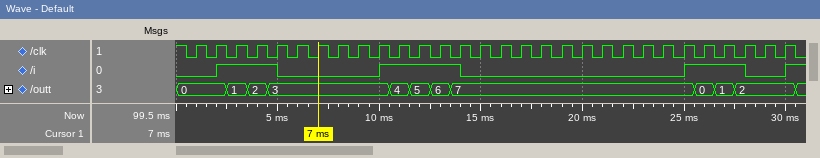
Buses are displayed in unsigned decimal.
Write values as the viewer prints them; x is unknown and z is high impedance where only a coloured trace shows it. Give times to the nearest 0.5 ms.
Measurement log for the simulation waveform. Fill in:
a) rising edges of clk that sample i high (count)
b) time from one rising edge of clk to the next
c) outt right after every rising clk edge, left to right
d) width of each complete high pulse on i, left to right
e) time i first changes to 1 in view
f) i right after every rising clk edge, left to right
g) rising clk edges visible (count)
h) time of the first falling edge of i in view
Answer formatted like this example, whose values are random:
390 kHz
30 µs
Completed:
10
1 ms
0, 0, 1, 2, 3, 3, 3, 3, 3, 3, 4, 5, 6, 7, 7, 7, 7, 7, 7, 7, 7, 7, 7, 7, 7, 0, 1, 2, 2, 2
3 ms, 4 ms, 3 ms
2 ms
0 1 1 1 0 0 0 0 0 1 1 1 1 0 0 0 0 0 0 0 0 0 0 0 1 1 1 0 0 1
30
5 ms
